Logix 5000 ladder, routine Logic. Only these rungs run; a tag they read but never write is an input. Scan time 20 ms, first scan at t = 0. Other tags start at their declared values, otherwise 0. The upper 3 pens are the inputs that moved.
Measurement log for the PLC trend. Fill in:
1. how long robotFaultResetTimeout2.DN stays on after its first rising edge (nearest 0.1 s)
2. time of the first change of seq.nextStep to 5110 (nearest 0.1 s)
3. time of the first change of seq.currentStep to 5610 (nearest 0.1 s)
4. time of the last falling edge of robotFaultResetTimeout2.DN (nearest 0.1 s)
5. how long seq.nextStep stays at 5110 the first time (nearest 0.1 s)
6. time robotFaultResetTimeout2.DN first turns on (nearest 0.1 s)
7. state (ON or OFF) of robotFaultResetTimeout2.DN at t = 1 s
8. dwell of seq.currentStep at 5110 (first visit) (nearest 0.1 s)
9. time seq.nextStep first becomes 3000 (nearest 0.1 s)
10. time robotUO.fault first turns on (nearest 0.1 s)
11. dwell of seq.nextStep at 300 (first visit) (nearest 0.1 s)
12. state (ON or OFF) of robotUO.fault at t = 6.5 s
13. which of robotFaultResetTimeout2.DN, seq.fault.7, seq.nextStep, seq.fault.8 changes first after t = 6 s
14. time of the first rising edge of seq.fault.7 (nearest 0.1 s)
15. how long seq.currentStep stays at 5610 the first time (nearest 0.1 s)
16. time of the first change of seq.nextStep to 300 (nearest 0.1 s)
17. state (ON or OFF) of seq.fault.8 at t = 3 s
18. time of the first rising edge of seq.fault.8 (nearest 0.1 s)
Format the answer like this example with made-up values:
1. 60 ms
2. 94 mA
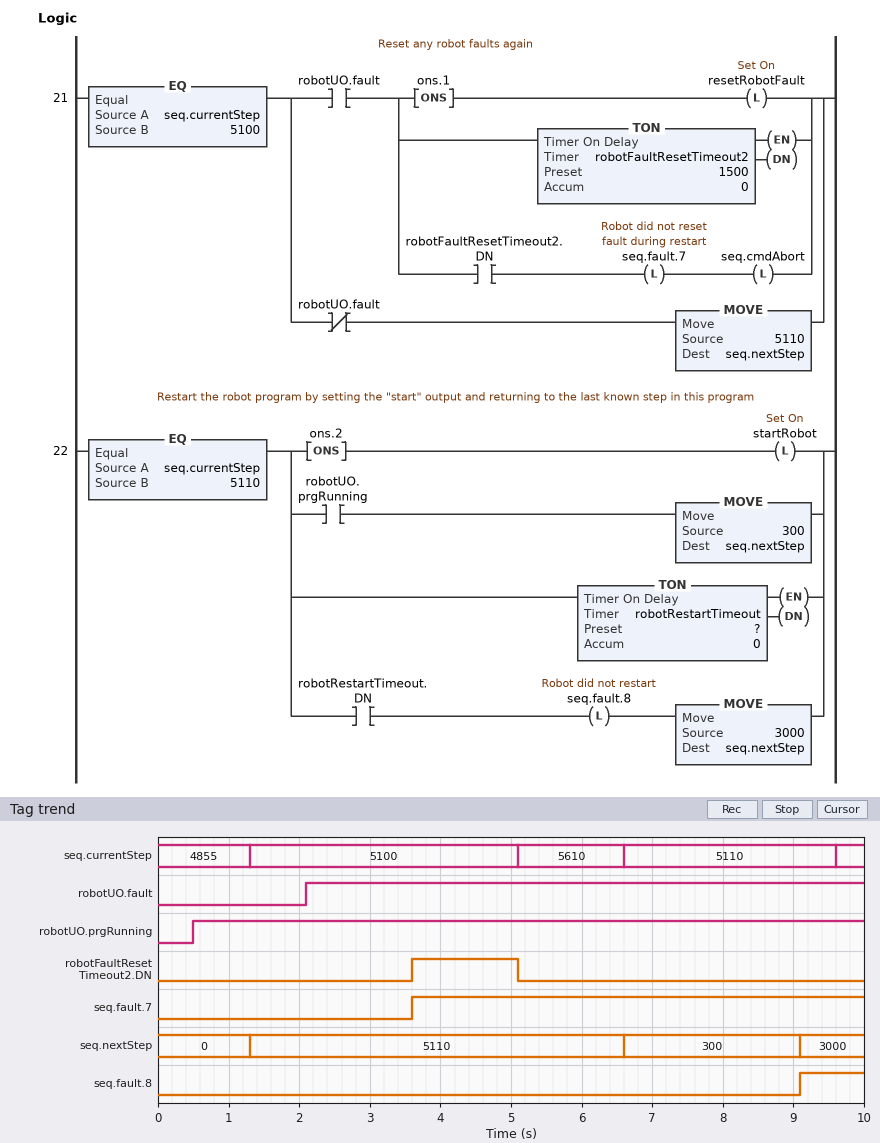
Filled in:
1. 1.5 s
2. 1.3 s
3. 5.1 s
4. 5.1 s
5. 5.3 s
6. 3.6 s
7. OFF
8. 3.0 s
9. 9.1 s
10. 2.1 s
11. 2.5 s
12. ON
13. seq.nextStep
14. 3.6 s
15. 1.5 s
16. 6.6 s
17. OFF
18. 9.1 s
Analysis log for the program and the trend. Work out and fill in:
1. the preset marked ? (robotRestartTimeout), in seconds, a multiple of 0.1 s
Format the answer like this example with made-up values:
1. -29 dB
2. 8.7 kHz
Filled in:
1. 2.5 s
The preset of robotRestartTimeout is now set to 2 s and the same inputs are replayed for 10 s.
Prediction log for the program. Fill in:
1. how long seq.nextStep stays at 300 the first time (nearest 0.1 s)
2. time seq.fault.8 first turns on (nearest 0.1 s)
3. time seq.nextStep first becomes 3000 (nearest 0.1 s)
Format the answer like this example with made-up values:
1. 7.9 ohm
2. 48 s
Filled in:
1. 2.0 s
2. 8.6 s
3. 8.6 s
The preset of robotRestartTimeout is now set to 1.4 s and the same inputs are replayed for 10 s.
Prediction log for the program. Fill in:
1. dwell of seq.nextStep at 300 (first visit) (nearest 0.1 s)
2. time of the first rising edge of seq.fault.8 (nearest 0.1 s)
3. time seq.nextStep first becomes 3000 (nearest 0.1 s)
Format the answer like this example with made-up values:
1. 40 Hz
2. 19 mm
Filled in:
1. 1.4 s
2. 8.0 s
3. 8.0 s
